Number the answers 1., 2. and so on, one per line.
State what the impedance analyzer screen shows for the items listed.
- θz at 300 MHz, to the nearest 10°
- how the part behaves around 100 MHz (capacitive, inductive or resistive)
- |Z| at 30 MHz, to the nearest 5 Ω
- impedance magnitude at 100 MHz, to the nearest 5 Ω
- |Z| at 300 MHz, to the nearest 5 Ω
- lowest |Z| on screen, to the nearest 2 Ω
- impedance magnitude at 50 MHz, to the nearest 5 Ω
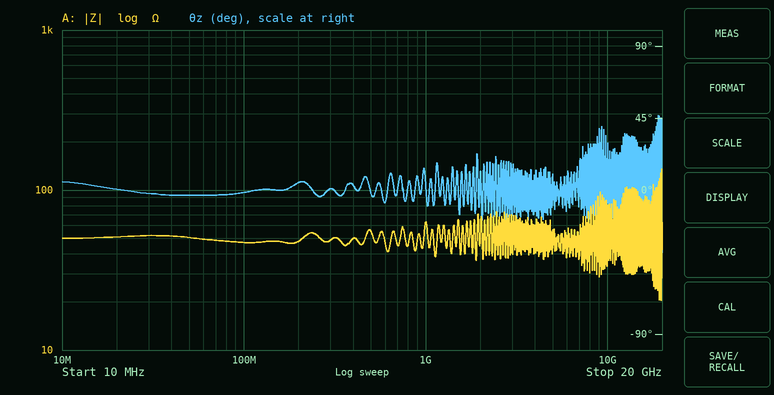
1. 0°
2. resistive
3. 50 Ω
4. 45 Ω
5. 50 Ω
6. 20 Ω
7. 50 Ω
